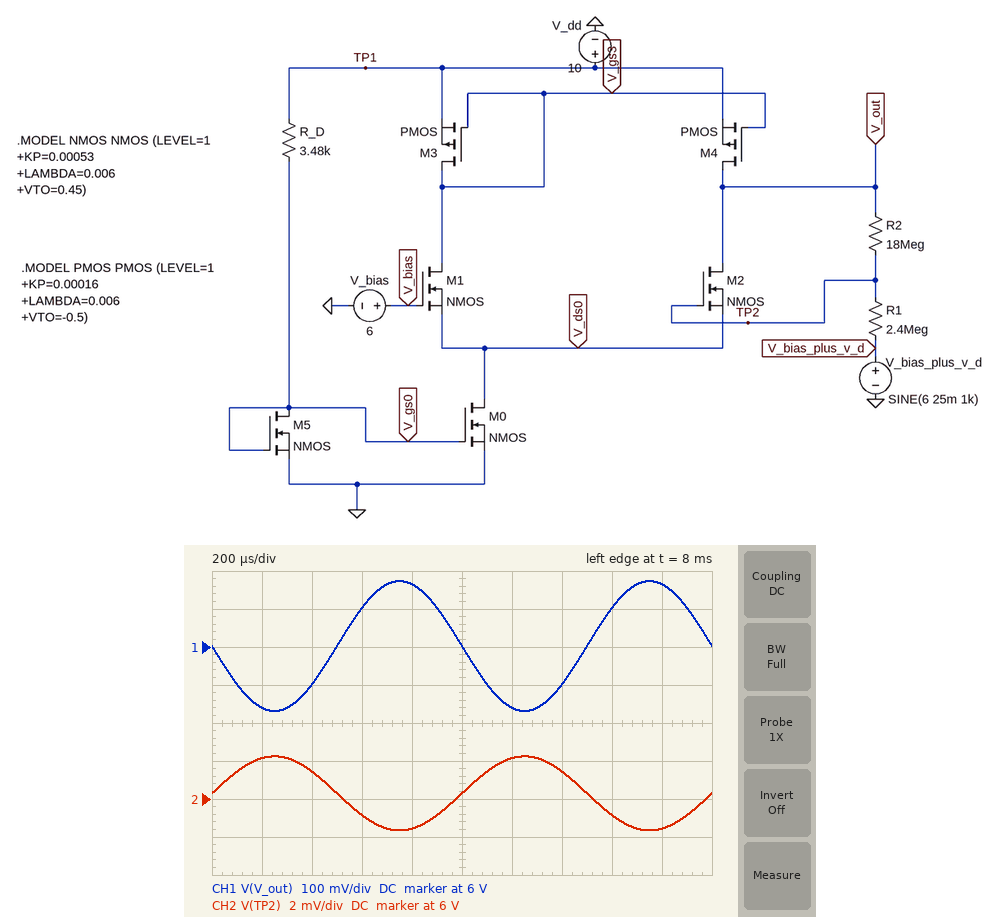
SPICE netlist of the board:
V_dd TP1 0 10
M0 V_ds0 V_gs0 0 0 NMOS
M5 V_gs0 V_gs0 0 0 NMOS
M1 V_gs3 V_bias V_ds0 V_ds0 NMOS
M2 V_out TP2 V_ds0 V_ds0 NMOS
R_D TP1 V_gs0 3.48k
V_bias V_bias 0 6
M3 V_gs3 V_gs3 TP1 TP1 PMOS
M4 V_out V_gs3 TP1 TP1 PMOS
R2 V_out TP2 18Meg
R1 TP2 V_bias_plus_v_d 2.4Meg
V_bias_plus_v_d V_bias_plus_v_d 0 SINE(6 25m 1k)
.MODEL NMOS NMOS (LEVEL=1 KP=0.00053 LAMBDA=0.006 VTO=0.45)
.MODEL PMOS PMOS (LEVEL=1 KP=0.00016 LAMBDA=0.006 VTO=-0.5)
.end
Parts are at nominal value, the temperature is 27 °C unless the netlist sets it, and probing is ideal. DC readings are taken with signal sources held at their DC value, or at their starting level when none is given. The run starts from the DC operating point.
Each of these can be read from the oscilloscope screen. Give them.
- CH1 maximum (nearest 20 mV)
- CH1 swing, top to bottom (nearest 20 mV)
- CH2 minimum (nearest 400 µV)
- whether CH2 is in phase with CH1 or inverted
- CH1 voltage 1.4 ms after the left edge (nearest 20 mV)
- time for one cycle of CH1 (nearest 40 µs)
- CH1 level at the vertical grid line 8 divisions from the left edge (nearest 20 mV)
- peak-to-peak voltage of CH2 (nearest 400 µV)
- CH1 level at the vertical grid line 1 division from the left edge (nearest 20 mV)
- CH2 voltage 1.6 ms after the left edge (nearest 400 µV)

6.18 V
340 mV
5.9984 V
inverted
5.90 V
1.00 ms
6.10 V
4.0 mV
5.84 V
5.9992 V
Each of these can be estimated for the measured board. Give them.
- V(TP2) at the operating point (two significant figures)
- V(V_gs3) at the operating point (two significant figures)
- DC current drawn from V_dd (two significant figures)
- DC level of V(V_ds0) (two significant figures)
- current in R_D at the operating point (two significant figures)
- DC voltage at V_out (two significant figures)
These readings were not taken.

6.0 V
6.0 V
3.9 mA
3.6 V
2.0 mA
6.0 V
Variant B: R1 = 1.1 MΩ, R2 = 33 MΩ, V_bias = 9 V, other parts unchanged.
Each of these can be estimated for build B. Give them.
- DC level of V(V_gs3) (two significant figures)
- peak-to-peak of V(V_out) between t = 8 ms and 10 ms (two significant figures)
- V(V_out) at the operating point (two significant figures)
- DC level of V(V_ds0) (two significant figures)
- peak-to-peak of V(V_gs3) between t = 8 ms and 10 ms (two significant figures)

5.2 V
31 mV
9.3 V
4.4 V
21 mV
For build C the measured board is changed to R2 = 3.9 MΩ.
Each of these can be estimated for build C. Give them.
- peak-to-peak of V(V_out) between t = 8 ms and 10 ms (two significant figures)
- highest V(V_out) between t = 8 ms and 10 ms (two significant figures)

79 mV
6.0 V
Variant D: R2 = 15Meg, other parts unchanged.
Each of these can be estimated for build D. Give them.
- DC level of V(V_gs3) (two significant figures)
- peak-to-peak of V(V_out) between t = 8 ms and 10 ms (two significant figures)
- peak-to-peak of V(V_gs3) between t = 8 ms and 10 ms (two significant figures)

6.0 V
290 mV
1.5 mV
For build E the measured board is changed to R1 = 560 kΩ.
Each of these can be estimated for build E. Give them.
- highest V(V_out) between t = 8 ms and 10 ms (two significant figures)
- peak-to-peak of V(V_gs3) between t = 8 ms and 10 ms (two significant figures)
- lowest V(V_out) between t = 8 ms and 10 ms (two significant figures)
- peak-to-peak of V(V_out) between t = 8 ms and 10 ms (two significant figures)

6.6 V
5.9 mV
5.5 V
1.1 V
